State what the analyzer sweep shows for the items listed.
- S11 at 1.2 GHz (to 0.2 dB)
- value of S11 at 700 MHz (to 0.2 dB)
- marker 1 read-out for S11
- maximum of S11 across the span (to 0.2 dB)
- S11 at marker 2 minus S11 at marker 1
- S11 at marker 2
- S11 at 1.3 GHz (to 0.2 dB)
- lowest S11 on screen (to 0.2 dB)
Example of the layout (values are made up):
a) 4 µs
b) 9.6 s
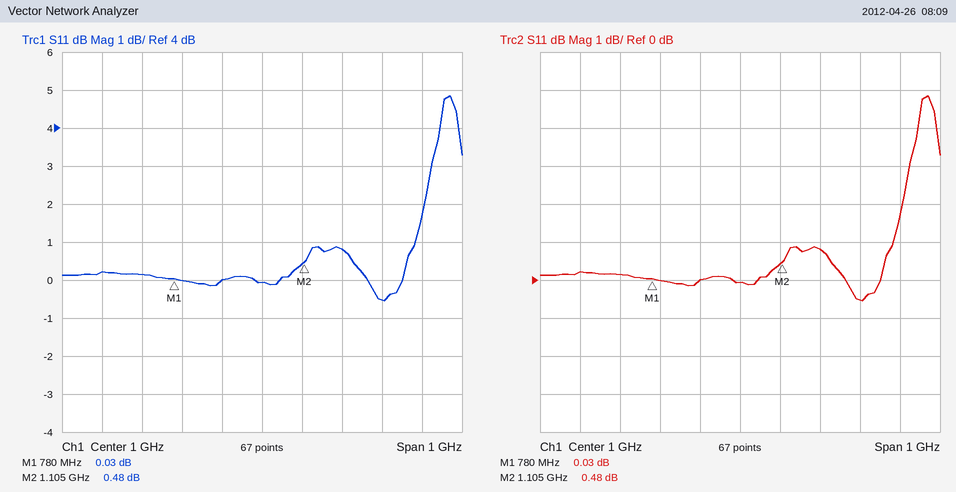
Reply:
a) 0.8 dB
b) 0.2 dB
c) 0.03 dB
d) 4.8 dB
e) 0.45 dB
f) 0.48 dB
g) -0.6 dB
h) -0.6 dB
